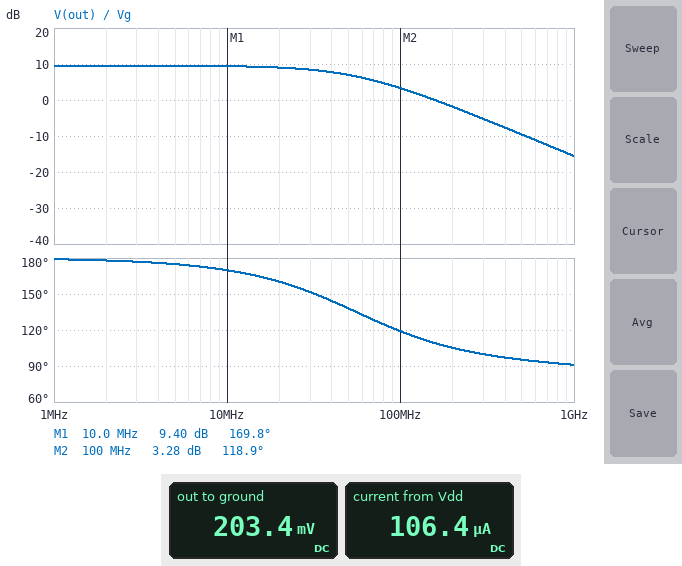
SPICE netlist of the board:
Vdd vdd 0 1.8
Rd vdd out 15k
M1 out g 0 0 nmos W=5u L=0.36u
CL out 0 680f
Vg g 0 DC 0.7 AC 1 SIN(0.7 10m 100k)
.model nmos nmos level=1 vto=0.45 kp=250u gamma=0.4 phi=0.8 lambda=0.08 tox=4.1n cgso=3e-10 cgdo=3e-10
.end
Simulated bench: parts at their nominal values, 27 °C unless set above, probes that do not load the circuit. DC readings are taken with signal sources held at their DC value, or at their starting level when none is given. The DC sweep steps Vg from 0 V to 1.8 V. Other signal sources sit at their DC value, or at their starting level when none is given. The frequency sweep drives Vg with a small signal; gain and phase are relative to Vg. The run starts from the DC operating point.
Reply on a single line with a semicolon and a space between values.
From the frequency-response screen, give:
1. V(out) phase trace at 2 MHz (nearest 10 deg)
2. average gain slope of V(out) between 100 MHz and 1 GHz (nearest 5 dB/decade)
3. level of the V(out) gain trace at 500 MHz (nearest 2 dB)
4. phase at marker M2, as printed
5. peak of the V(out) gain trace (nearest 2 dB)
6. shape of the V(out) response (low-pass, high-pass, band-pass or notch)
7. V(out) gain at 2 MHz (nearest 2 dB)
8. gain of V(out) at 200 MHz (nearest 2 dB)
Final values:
180 deg; -20 dB/decade; -10 dB; 118.9 deg; 10 dB; low-pass; 10 dB; -2 dB
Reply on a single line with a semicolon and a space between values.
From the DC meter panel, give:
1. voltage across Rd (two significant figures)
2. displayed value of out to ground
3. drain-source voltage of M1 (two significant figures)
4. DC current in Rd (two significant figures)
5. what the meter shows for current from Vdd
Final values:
1.6 V; 203.4 mV; 200 mV; 110 µA; 106.4 µA
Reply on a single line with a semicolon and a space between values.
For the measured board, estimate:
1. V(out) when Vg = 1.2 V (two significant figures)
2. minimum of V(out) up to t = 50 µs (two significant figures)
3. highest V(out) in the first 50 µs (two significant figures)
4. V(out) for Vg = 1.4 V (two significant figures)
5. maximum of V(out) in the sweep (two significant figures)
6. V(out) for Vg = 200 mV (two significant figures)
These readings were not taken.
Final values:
46 mV; 180 mV; 270 mV; 36 mV; 1.8 V; 1.8 V
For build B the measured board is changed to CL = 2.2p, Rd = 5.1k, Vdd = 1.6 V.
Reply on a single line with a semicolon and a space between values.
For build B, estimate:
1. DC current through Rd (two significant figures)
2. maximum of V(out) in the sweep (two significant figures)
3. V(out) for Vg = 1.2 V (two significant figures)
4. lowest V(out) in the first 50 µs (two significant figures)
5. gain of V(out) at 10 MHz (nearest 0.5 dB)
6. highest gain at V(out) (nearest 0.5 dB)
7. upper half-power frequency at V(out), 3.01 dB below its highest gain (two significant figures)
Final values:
120 µA; 1.6 V; 120 mV; 960 mV; 11.5 dB; 13.0 dB; 15 MHz
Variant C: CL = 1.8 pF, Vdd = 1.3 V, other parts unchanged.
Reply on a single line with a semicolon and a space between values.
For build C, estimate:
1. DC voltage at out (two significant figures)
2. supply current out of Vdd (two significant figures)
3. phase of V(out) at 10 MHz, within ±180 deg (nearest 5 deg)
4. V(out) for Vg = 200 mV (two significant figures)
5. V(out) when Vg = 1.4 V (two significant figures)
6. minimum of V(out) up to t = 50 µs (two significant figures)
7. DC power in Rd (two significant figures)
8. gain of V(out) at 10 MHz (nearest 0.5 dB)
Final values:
120 mV; 79 µA; 170 deg; 1.3 V; 26 mV; 110 mV; 93 µW; -2.5 dB
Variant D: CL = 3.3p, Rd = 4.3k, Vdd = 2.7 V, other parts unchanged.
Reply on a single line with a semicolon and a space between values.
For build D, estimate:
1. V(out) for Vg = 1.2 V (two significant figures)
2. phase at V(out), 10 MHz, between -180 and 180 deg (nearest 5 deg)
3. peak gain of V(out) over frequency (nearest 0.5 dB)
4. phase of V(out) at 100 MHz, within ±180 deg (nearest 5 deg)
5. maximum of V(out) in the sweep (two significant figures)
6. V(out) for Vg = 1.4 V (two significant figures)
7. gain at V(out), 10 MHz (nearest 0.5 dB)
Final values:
260 mV; 140 deg; 12.5 dB; 95 deg; 2.7 V; 190 mV; 10.0 dB
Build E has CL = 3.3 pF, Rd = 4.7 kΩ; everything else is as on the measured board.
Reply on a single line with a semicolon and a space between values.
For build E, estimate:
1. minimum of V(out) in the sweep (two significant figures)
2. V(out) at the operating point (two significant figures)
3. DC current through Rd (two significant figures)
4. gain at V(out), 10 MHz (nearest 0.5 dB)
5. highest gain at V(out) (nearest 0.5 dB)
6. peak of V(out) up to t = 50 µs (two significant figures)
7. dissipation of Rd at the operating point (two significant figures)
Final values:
80 mV; 1.2 V; 120 µA; 10.0 dB; 12.5 dB; 1.3 V; 67 µW
